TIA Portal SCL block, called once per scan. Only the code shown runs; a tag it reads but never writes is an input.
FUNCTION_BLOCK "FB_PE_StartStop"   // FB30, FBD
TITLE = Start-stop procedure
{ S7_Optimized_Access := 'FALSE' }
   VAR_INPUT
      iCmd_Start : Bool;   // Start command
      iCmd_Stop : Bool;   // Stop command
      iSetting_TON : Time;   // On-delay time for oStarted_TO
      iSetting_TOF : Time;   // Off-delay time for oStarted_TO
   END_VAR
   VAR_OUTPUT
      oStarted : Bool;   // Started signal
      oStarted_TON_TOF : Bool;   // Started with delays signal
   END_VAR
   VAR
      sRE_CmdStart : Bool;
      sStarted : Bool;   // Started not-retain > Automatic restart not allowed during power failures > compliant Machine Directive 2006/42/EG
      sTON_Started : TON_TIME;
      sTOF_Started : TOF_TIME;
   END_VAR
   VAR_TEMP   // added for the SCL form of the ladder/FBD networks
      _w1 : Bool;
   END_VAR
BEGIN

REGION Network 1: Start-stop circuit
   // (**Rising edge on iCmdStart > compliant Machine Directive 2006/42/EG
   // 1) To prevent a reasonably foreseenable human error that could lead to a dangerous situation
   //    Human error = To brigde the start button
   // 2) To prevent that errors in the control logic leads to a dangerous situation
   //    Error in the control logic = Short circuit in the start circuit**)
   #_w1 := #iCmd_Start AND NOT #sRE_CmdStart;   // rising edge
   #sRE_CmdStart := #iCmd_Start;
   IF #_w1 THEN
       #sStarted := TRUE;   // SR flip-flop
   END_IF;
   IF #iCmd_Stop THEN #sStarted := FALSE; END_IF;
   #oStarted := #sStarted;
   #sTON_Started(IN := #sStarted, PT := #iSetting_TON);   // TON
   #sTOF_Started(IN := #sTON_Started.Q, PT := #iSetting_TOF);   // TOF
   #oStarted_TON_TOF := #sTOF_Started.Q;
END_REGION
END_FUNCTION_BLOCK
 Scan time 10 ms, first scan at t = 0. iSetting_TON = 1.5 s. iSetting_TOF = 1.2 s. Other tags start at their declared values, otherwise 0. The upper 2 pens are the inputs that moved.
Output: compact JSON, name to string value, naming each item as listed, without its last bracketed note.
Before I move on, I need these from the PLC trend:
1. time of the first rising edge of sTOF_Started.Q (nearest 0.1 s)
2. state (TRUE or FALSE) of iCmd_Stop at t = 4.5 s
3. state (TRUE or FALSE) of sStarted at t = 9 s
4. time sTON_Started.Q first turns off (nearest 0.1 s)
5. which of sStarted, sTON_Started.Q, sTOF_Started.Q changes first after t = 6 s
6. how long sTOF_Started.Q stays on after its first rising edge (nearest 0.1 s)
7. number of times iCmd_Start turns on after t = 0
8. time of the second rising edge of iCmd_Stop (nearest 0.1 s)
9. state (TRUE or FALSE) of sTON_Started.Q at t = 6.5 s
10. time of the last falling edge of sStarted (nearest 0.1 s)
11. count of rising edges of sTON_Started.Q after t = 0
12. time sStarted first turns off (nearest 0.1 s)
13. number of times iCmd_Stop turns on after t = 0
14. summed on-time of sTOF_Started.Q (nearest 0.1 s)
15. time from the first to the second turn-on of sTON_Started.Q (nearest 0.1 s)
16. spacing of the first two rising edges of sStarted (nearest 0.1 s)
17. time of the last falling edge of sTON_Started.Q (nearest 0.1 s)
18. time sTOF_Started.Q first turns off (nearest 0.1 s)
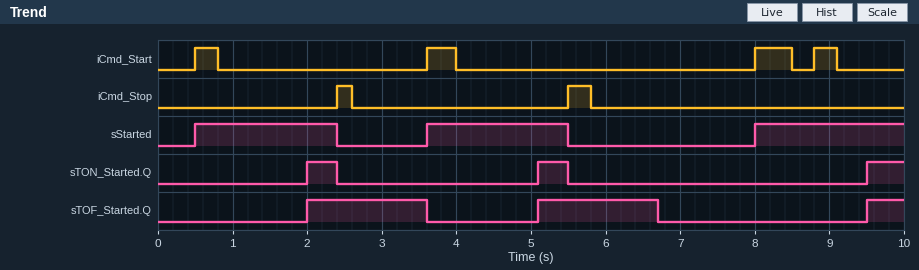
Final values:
{"time of the first rising edge of sTOF_Started.Q": "2.0 s", "state (TRUE or FALSE) of iCmd_Stop at t = 4.5 s": "FALSE", "state (TRUE or FALSE) of sStarted at t = 9 s": "TRUE", "time sTON_Started.Q first turns off": "2.4 s", "which of sStarted, sTON_Started.Q, sTOF_Started.Q changes first after t = 6 s": "sTOF_Started.Q", "how long sTOF_Started.Q stays on after its first rising edge": "1.6 s", "number of times iCmd_Start turns on after t = 0": "4", "time of the second rising edge of iCmd_Stop": "5.5 s", "state (TRUE or FALSE) of sTON_Started.Q at t = 6.5 s": "FALSE", "time of the last falling edge of sStarted": "5.5 s", "count of rising edges of sTON_Started.Q after t = 0": "3", "time sStarted first turns off": "2.4 s", "number of times iCmd_Stop turns on after t = 0": "2", "summed on-time of sTOF_Started.Q": "3.7 s", "time from the first to the second turn-on of sTON_Started.Q": "3.1 s", "spacing of the first two rising edges of sStarted": "3.1 s", "time of the last falling edge of sTON_Started.Q": "5.5 s", "time sTOF_Started.Q first turns off": "3.6 s"}
